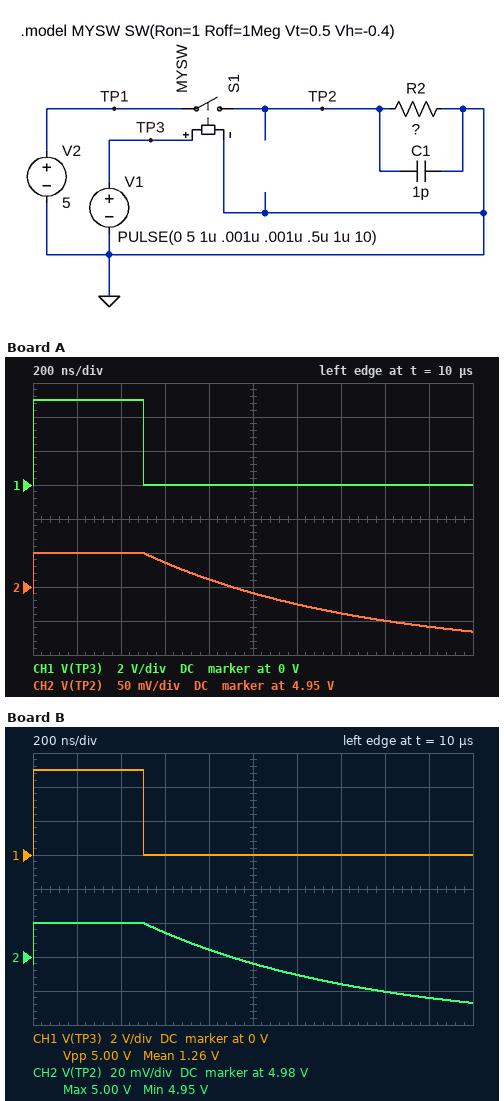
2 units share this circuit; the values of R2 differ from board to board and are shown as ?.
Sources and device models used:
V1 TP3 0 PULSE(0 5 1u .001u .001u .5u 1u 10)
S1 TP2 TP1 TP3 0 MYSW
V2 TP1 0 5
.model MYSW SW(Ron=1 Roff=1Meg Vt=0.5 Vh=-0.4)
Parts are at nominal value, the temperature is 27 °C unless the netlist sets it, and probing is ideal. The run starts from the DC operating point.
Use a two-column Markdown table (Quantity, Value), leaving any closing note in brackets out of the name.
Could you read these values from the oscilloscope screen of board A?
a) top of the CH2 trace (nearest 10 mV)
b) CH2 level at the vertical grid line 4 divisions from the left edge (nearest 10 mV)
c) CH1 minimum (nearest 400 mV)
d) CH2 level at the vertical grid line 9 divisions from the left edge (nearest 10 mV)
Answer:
| Quantity | Value |
|---|---|
| top of the CH2 trace | 5.00 V |
| CH2 level at the vertical grid line 4 divisions from the left edge | 4.96 V |
| CH1 minimum | 0 V |
| CH2 level at the vertical grid line 9 divisions from the left edge | 4.89 V |
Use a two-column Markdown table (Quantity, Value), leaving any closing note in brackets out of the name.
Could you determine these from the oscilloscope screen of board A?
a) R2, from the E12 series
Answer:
| Quantity | Value |
|---|---|
| R2, from the E12 series | 33 MΩ |
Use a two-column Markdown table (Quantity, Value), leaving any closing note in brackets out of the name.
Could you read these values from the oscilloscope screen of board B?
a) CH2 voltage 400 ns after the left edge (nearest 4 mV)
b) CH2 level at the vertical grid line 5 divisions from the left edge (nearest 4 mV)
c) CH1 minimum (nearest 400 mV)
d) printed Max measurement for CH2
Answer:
| Quantity | Value |
|---|---|
| CH2 voltage 400 ns after the left edge | 5.000 V |
| CH2 level at the vertical grid line 5 divisions from the left edge | 4.976 V |
| CH1 minimum | 0 V |
| printed Max measurement for CH2 | 5.00 V |
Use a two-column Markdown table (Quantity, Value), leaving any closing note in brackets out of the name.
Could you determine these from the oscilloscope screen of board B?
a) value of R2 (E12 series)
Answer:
| Quantity | Value |
|---|---|
| value of R2 | 82 MΩ |
